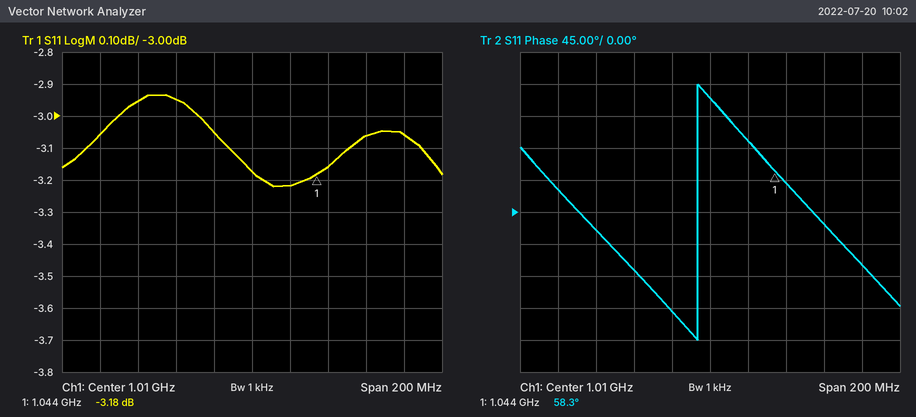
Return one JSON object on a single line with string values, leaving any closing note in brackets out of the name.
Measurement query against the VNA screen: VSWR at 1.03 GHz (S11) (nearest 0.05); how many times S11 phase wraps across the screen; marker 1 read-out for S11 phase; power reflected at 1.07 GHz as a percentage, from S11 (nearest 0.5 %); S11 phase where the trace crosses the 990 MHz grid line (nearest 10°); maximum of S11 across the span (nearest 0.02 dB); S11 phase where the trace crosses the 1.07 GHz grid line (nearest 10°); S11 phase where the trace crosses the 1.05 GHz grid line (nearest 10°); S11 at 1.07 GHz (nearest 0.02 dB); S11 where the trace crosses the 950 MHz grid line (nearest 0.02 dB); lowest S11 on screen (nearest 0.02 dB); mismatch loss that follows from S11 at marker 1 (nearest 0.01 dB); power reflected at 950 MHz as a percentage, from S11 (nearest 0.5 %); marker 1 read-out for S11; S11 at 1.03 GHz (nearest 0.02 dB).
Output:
{"VSWR at 1.03 GHz (S11)": "5.45", "how many times S11 phase wraps across the screen": "1", "marker 1 read-out for S11 phase": "58.3°", "power reflected at 1.07 GHz as a percentage, from S11": "49.5 %", "S11 phase where the trace crosses the 990 MHz grid line": "-140°", "maximum of S11 across the span": "-2.94 dB", "S11 phase where the trace crosses the 1.07 GHz grid line": "-20°", "S11 phase where the trace crosses the 1.05 GHz grid line": "40°", "S11 at 1.07 GHz": "-3.06 dB", "S11 where the trace crosses the 950 MHz grid line": "-2.96 dB", "lowest S11 on screen": "-3.22 dB", "mismatch loss that follows from S11 at marker 1": "2.85 dB", "power reflected at 950 MHz as a percentage, from S11": "50.5 %", "marker 1 read-out for S11": "-3.18 dB", "S11 at 1.03 GHz": "-3.22 dB"}
